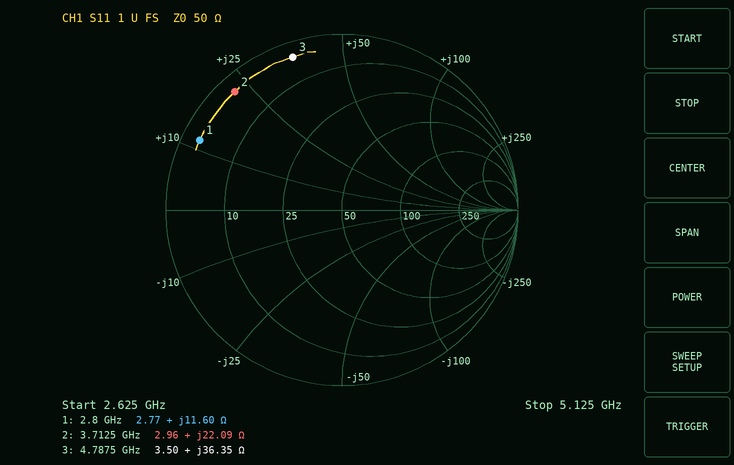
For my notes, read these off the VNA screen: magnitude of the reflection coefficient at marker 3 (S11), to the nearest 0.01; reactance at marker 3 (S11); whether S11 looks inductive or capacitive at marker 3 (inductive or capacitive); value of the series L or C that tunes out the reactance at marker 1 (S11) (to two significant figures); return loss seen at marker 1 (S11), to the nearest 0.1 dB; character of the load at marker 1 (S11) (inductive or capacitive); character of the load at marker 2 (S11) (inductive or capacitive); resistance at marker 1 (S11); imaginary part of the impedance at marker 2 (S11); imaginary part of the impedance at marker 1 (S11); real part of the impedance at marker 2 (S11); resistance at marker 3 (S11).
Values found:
0.91
+36.35 Ω
inductive
4.9 pF
0.9 dB
inductive
inductive
2.77 Ω
+22.09 Ω
+11.60 Ω
2.96 Ω
3.50 Ω
